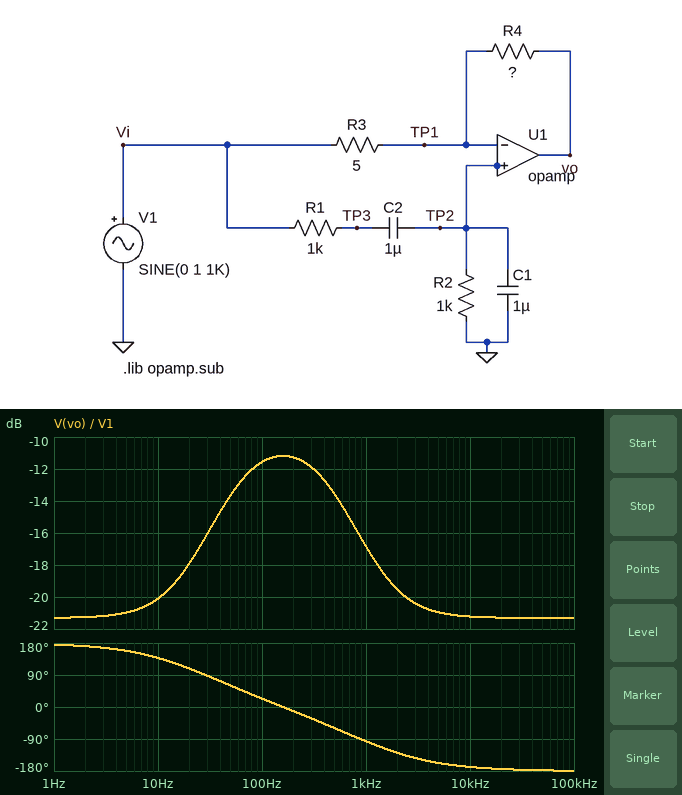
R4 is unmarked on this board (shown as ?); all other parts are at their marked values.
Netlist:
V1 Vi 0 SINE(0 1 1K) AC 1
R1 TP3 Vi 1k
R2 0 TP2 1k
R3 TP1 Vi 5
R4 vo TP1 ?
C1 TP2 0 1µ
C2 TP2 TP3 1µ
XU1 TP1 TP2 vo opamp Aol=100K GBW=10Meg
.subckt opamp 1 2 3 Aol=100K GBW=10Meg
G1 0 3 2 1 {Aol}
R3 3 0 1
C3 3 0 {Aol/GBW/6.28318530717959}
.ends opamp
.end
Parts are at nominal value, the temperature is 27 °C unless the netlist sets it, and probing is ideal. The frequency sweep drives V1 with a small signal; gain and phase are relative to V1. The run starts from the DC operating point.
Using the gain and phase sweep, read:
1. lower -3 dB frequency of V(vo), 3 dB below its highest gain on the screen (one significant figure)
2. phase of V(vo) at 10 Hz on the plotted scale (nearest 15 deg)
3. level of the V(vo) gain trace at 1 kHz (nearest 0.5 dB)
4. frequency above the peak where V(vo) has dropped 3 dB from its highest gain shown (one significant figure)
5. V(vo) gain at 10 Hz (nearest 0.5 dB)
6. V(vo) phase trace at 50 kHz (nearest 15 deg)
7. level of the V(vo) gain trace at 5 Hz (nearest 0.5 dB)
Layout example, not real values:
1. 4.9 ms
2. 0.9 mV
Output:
1. 40 Hz
2. 135 deg
3. -17.0 dB
4. 600 Hz
5. -20.0 dB
6. -180 deg
7. -21.0 dB
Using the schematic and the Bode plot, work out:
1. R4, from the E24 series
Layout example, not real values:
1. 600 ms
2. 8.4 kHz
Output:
1. 0.43 Ω
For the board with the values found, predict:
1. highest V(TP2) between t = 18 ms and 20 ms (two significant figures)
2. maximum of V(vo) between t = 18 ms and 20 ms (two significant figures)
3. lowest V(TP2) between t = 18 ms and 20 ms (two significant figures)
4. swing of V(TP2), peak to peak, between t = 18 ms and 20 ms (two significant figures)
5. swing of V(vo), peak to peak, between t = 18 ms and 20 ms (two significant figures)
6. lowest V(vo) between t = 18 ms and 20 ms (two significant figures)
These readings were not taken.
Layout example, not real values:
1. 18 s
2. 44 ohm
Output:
1. 150 mV
2. 140 mV
3. -150 mV
4. 290 mV
5. 290 mV
6. -140 mV
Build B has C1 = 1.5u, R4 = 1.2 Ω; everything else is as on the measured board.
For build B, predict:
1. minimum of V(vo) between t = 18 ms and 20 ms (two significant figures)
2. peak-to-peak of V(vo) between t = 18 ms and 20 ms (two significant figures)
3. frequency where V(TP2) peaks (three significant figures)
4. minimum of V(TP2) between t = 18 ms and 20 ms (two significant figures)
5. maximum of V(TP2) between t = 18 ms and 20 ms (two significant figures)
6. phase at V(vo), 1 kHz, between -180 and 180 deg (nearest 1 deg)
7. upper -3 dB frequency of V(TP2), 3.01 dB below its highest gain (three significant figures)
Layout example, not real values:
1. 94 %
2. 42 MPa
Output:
1. -230 mV
2. 460 mV
3. 130 Hz
4. -100 mV
5. 100 mV
6. -149 deg
7. 412 Hz
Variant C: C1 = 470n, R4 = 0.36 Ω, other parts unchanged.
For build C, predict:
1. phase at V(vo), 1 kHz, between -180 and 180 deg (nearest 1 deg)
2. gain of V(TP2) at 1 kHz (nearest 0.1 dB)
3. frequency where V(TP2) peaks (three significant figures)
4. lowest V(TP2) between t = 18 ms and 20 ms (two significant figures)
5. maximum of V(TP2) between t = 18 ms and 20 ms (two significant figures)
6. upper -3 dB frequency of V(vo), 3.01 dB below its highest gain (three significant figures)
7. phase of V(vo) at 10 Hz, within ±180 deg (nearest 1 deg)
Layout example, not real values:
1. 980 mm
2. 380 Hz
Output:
1. -61 deg
2. -11.4 dB
3. 232 Hz
4. -270 mV
5. 270 mV
6. 930 Hz
7. 133 deg
